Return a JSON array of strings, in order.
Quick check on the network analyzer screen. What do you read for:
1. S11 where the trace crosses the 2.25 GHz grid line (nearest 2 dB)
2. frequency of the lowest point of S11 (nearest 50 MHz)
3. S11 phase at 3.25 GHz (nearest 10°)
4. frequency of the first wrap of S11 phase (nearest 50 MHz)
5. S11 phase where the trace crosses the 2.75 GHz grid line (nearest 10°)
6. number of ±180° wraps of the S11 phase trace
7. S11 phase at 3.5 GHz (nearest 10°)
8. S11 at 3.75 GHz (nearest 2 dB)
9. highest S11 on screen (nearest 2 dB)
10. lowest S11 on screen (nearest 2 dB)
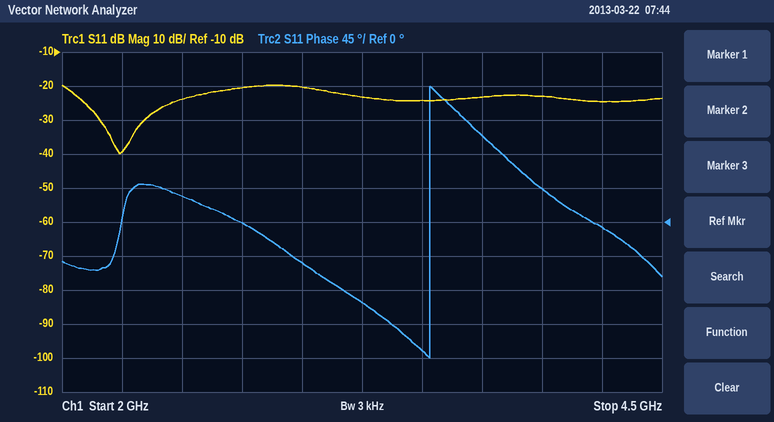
["-40 dB", "2.25 GHz", "-110°", "3.55 GHz", "0°", "1", "-170°", "-24 dB", "-20 dB", "-40 dB"]
